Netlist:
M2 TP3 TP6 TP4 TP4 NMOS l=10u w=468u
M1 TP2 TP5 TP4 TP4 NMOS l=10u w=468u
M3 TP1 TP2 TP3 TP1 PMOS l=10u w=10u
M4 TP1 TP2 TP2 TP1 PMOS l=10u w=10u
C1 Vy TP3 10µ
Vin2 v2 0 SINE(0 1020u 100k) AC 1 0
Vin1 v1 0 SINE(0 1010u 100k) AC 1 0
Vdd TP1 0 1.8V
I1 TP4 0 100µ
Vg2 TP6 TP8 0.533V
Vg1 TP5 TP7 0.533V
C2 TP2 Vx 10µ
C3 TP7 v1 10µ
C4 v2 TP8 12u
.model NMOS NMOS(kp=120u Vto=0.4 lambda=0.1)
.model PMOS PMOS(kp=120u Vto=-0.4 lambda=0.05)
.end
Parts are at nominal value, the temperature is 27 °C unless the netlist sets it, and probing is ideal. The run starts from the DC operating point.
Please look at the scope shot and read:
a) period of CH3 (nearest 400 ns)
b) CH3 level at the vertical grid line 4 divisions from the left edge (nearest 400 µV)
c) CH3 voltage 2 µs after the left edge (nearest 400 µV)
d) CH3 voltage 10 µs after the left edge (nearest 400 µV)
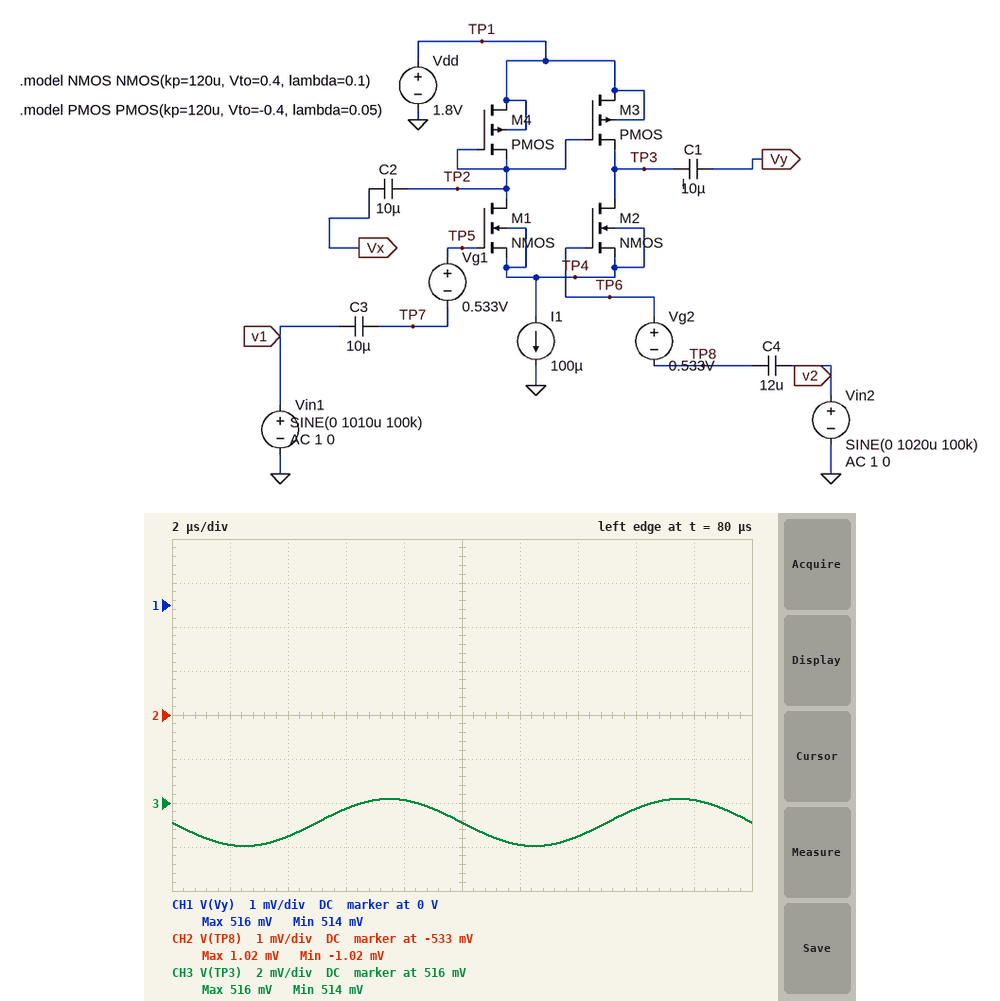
10.0 µs
516.0 mV
514.0 mV
515.2 mV
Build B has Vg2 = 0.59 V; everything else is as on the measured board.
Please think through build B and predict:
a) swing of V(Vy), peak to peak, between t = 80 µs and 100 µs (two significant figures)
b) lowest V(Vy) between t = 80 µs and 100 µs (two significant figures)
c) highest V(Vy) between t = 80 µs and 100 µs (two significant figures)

2.0 mV
59 mV
61 mV
